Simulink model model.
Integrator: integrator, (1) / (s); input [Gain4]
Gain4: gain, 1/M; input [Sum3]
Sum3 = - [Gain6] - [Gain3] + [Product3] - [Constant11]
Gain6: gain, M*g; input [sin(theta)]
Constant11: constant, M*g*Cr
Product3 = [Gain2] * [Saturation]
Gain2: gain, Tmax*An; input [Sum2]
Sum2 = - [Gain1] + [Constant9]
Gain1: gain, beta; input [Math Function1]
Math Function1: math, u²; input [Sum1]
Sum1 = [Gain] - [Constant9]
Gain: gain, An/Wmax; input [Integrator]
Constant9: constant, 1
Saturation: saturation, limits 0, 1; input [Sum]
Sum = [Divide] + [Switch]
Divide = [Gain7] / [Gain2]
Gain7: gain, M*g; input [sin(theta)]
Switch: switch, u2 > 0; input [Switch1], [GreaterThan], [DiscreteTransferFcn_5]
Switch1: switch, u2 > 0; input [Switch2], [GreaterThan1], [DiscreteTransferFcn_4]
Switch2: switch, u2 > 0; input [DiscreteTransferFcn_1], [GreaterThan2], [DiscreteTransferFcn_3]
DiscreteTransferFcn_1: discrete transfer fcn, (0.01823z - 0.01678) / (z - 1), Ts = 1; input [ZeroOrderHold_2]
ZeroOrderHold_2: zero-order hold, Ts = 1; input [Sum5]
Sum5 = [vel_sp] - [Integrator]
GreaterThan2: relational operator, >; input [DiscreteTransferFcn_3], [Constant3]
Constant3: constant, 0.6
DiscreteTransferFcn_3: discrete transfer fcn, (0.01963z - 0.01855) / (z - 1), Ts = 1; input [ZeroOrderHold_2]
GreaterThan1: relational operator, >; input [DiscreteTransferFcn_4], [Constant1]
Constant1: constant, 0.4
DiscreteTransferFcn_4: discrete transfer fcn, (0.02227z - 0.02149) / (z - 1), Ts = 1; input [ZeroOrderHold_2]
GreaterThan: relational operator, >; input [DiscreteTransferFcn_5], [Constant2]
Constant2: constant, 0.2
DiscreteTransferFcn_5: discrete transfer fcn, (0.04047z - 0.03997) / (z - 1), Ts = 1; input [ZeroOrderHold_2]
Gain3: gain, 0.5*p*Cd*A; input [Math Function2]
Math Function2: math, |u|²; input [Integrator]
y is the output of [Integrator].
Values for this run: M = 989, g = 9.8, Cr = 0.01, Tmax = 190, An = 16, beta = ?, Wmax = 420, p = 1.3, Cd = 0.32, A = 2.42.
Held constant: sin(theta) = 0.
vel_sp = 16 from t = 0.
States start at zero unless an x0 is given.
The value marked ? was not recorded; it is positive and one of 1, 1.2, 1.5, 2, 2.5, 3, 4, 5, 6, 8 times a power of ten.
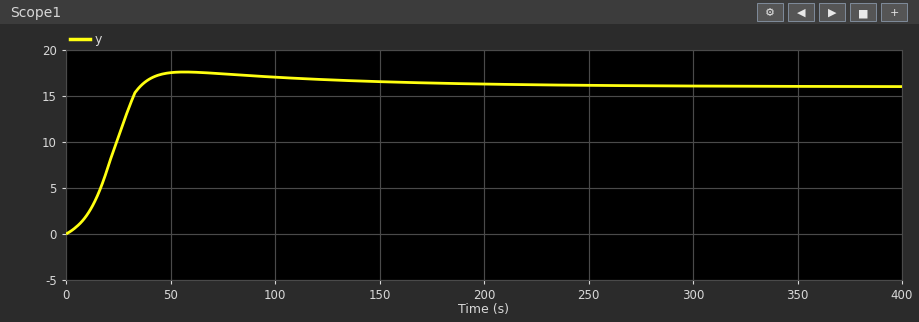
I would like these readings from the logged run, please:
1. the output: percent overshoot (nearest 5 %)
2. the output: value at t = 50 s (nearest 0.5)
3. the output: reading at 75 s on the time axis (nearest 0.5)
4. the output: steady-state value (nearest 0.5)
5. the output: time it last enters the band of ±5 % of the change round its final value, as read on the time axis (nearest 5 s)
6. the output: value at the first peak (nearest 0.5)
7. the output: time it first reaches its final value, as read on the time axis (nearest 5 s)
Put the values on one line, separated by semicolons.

10 %; 17.5; 17.5; 16.0; 120 s; 17.5; 35 s
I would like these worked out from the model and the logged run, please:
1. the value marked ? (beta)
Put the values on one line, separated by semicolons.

0.8
